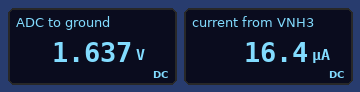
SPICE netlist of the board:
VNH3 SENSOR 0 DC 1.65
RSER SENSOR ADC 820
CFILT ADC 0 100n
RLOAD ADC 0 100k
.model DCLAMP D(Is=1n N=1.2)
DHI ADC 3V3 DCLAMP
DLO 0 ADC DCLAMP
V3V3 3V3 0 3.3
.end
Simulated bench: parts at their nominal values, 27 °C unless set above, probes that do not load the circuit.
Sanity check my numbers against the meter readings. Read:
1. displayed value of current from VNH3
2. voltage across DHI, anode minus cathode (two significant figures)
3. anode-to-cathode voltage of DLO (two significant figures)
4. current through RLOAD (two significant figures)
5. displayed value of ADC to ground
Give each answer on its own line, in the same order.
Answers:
16.4 µA
-1.7 V
-1.6 V
16 µA
1.637 V
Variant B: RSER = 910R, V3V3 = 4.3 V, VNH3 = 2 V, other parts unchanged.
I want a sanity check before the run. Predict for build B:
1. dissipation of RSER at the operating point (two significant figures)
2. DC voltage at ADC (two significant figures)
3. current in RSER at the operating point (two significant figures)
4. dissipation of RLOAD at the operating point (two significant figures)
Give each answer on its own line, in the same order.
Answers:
360 nW
2.0 V
20 µA
39 µW
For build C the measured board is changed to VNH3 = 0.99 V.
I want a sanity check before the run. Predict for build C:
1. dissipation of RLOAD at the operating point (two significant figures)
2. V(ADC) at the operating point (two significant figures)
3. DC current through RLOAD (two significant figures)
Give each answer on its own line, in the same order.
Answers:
9.6 µW
980 mV
9.8 µA
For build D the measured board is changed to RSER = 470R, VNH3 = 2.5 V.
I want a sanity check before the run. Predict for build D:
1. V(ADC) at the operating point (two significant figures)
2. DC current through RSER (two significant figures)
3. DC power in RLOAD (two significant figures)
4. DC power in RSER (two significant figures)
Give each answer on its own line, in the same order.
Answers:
2.5 V
25 µA
62 µW
290 nW
